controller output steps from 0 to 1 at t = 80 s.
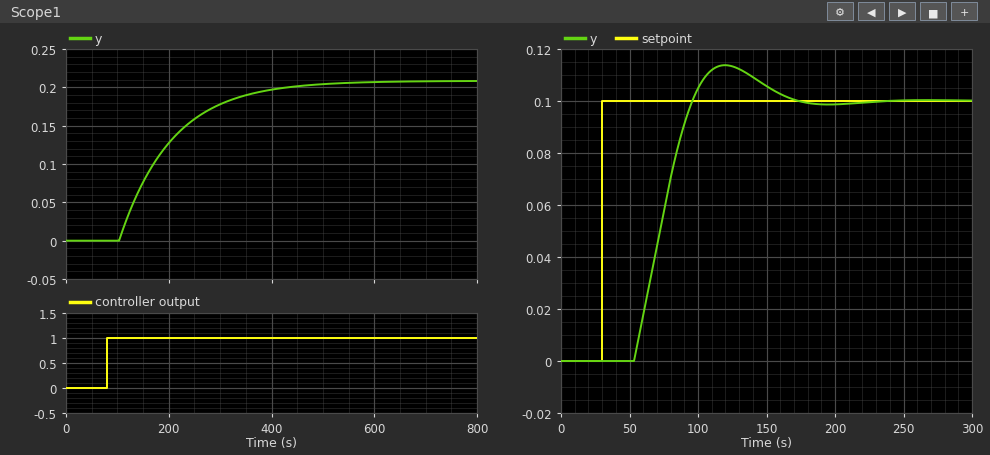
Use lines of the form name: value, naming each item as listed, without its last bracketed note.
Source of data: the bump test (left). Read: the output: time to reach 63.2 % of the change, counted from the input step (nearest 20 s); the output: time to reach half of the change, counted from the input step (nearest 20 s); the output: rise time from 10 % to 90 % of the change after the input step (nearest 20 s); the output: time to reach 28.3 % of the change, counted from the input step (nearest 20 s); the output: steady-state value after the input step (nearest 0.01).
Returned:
the output: time to reach 63.2 % of the change, counted from the input step: 120 s
the output: time to reach half of the change, counted from the input step: 100 s
the output: rise time from 10 % to 90 % of the change after the input step: 220 s
the output: time to reach 28.3 % of the change, counted from the input step: 60 s
the output: steady-state value after the input step: 0.21
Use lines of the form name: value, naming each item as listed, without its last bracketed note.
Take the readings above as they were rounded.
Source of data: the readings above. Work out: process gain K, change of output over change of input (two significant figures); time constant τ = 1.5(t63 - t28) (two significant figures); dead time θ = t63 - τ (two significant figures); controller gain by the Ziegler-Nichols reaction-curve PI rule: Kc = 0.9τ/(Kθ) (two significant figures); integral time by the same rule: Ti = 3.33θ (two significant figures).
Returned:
process gain K, change of output over change of input: 0.21
time constant τ = 1.5(t63 - t28): 90 s
dead time θ = t63 - τ: 30 s
controller gain by the Ziegler-Nichols reaction-curve PI rule: Kc = 0.9τ/(Kθ): 13
integral time by the same rule: Ti = 3.33θ: 100 s
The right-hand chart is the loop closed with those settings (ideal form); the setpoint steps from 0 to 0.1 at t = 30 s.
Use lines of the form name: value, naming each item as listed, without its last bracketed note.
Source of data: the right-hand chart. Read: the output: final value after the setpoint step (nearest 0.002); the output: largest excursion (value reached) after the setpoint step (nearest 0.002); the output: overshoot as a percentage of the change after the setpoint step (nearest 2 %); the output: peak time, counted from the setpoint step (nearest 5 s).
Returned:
the output: final value after the setpoint step: 0.100
the output: largest excursion (value reached) after the setpoint step: 0.114
the output: overshoot as a percentage of the change after the setpoint step: 14 %
the output: peak time, counted from the setpoint step: 90 s
